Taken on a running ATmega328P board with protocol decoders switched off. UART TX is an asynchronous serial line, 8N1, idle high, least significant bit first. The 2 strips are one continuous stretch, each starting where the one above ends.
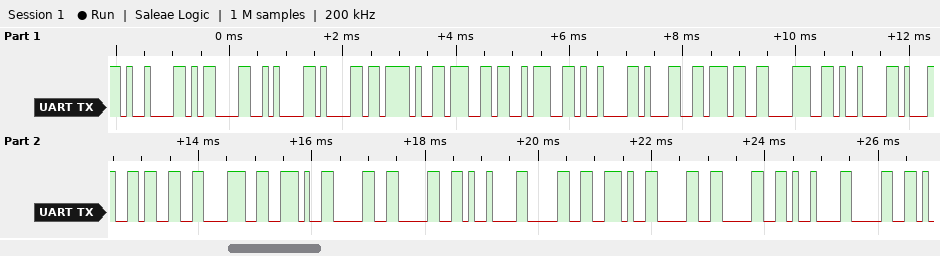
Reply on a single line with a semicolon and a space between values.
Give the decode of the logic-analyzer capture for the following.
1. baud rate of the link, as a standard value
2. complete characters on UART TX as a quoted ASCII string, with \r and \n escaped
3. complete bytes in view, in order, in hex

9600 baud; "\t\r\na/g:\t178\t138.00\t0.00\t0"; 09 0D 0A 61 2F 67 3A 09 31 37 38 09 31 33 38 2E 30 30 09 30 2E 30 30 09 30
